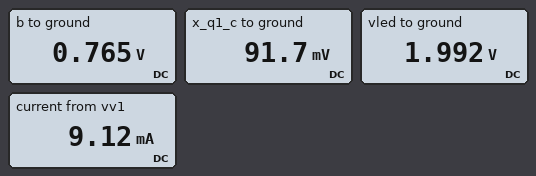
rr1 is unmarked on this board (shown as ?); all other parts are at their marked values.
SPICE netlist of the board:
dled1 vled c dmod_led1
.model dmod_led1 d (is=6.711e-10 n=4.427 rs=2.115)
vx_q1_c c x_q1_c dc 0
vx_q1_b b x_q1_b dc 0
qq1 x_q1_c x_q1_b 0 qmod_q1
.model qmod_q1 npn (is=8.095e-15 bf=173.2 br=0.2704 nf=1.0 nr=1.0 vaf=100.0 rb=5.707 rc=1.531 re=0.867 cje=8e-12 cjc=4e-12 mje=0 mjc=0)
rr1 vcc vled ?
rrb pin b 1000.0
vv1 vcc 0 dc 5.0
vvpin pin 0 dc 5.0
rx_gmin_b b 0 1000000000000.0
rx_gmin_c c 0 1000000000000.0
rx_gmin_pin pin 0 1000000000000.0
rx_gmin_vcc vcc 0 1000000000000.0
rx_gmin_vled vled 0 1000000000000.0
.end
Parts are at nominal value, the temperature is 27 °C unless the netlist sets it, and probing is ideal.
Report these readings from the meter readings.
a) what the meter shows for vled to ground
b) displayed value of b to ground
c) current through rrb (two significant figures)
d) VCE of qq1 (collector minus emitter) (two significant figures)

1.992 V
0.765 V
4.2 mA
92 mV
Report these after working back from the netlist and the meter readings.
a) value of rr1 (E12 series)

330 Ω
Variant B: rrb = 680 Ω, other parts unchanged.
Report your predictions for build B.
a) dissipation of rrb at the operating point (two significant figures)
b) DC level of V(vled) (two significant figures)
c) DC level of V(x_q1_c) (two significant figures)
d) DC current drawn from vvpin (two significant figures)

26 mW
2.0 V
88 mV
6.2 mA
